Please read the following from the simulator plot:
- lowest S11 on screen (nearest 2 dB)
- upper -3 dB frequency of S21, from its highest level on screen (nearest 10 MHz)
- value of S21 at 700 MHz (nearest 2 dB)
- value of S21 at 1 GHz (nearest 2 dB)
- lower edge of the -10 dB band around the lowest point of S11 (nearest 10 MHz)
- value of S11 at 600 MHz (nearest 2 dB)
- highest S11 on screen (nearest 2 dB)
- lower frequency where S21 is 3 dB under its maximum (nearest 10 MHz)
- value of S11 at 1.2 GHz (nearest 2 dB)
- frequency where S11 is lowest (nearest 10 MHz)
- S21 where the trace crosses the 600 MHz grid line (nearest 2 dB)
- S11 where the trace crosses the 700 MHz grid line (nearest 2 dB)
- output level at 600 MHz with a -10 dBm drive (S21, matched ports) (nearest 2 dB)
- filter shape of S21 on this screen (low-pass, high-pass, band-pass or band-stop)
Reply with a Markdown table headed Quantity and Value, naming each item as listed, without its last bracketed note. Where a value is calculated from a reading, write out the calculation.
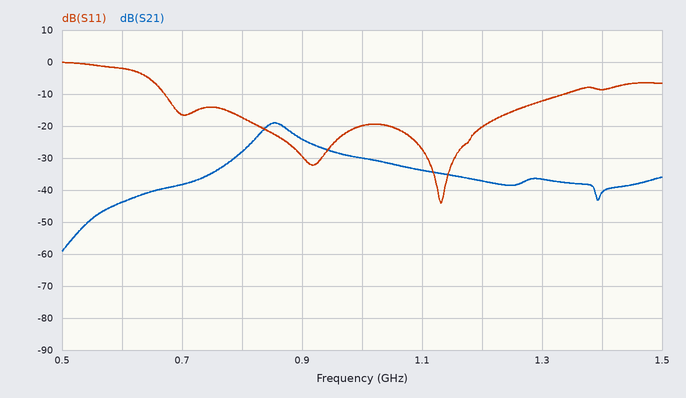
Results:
| Quantity | Value |
|---|---|
| lowest S11 on screen | -44 dB |
| upper -3 dB frequency of S21, from its highest level on screen | 880 MHz |
| value of S21 at 700 MHz | -38 dB |
| value of S21 at 1 GHz | -30 dB |
| lower edge of the -10 dB band around the lowest point of S11 | 670 MHz |
| value of S11 at 600 MHz | -2 dB |
| highest S11 on screen | 0 dB |
| lower frequency where S21 is 3 dB under its maximum | 830 MHz |
| value of S11 at 1.2 GHz | -20 dB |
| frequency where S11 is lowest | 1.13 GHz |
| S21 where the trace crosses the 600 MHz grid line | -44 dB |
| S11 where the trace crosses the 700 MHz grid line | -16 dB |
| output level at 600 MHz with a -10 dBm drive (S21, matched ports) | -10 dBm + (-44 dB) = -54 dBm |
| filter shape of S21 on this screen | band-pass |
